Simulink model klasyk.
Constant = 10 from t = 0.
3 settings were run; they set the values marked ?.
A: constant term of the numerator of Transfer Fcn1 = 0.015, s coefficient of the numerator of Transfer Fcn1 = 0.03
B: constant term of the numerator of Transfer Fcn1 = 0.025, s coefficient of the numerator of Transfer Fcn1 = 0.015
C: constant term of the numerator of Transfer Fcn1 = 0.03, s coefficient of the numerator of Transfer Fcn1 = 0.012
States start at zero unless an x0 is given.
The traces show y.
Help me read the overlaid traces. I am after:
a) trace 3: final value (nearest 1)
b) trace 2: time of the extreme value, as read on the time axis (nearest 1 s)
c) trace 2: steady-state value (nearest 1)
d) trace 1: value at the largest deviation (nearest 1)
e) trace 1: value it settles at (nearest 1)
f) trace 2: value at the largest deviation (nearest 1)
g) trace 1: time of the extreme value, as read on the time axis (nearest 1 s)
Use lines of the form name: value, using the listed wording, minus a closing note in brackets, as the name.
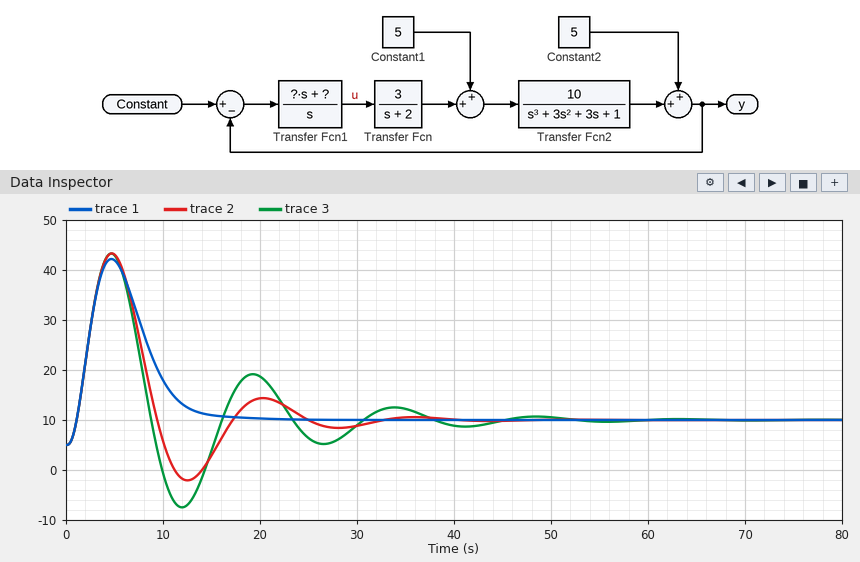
trace 3: final value: 10
trace 2: time of the extreme value, as read on the time axis: 5 s
trace 2: steady-state value: 10
trace 1: value at the largest deviation: 42
trace 1: value it settles at: 10
trace 2: value at the largest deviation: 43
trace 1: time of the extreme value, as read on the time axis: 5 s
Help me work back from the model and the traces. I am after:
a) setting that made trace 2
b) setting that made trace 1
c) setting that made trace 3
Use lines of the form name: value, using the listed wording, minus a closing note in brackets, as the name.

setting that made trace 2: B
setting that made trace 1: A
setting that made trace 3: C
